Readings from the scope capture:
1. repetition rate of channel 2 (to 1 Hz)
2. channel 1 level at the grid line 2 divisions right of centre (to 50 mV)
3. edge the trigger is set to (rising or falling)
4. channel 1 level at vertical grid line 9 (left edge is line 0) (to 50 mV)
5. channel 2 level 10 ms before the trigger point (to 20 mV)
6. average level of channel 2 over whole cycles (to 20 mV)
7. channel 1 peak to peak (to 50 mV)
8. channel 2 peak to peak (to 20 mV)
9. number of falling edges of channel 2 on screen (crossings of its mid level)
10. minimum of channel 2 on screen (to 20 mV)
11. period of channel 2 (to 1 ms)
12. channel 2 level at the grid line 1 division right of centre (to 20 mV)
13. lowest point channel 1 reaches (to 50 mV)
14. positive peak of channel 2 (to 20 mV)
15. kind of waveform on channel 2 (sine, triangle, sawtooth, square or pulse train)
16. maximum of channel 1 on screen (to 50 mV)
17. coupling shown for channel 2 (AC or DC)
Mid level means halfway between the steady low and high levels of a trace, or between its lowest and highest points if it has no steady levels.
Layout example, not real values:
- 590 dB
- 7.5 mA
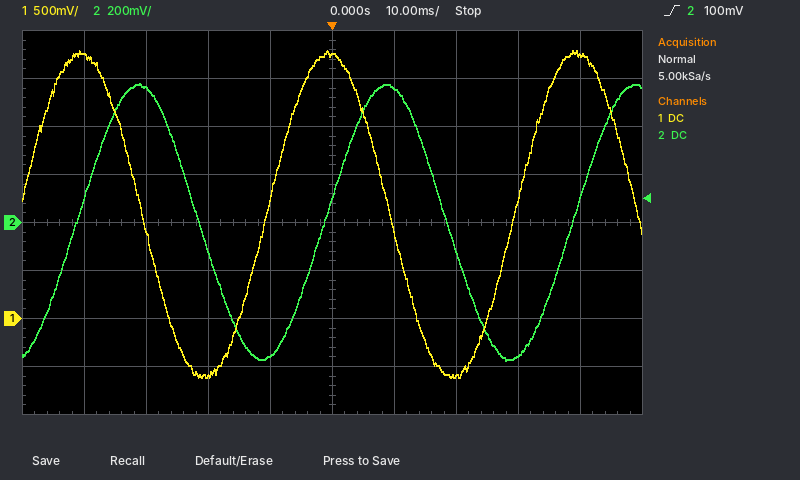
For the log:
- 25 Hz
- -600 mV
- rising
- 2.75 V
- -560 mV
- 0 mV
- 3.40 V
- 1.16 V
- 2
- -580 mV
- 40 ms
- 560 mV
- -600 mV
- 580 mV
- sine
- 2.80 V
- DC
